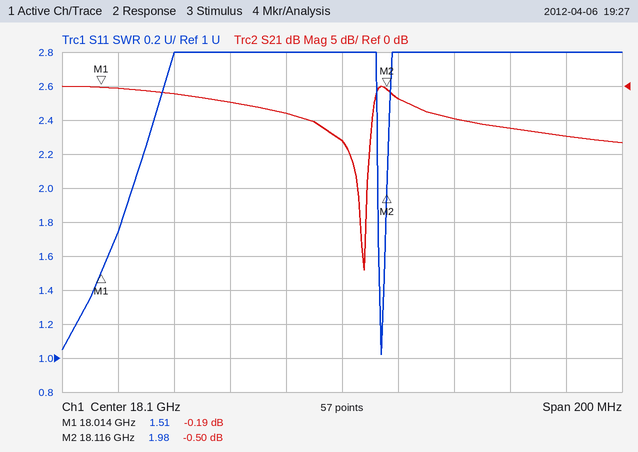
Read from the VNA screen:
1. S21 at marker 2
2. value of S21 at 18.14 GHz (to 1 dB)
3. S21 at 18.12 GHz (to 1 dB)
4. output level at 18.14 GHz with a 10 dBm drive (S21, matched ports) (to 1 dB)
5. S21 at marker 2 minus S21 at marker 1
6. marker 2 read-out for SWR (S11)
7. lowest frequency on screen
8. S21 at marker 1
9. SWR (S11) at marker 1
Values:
-0.50 dB
-5 dB
-2 dB
5 dBm
-0.31 dB
1.98
18 GHz
-0.19 dB
1.51
